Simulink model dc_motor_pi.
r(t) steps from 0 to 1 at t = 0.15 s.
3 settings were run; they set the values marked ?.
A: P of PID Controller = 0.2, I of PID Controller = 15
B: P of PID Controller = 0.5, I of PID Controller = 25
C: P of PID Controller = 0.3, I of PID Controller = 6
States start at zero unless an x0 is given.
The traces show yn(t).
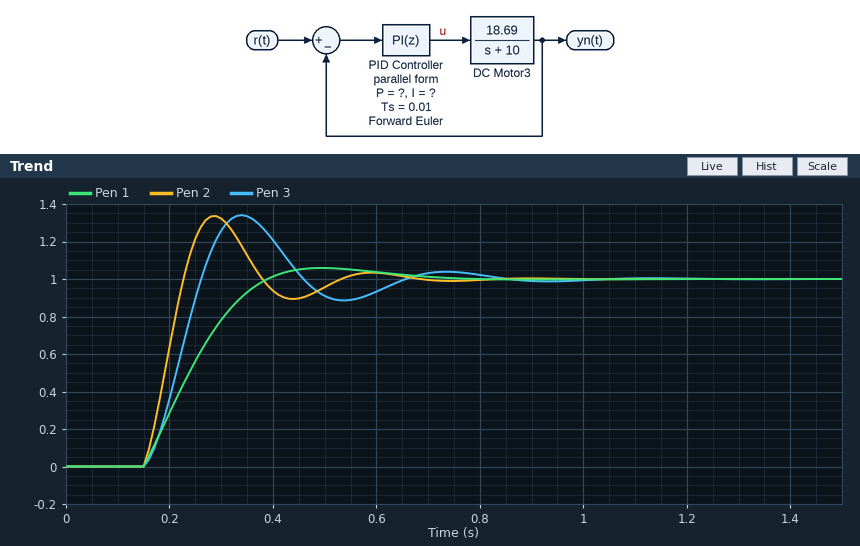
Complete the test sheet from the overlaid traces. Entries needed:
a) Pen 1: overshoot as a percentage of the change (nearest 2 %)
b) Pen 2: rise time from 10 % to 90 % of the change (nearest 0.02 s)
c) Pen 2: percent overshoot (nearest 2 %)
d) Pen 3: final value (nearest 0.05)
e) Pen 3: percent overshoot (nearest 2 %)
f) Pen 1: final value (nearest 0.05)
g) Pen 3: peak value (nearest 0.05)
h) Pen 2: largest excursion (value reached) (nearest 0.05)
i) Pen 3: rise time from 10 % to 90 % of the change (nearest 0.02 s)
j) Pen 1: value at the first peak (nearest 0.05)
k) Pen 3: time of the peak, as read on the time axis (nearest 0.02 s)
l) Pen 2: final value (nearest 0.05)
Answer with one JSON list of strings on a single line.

["6 %", "0.06 s", "34 %", "1.00", "34 %", "1.00", "1.35", "1.35", "0.08 s", "1.05", "0.34 s", "1.00"]
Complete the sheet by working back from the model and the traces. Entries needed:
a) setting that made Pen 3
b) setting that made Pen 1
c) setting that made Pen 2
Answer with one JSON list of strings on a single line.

["A", "C", "B"]
